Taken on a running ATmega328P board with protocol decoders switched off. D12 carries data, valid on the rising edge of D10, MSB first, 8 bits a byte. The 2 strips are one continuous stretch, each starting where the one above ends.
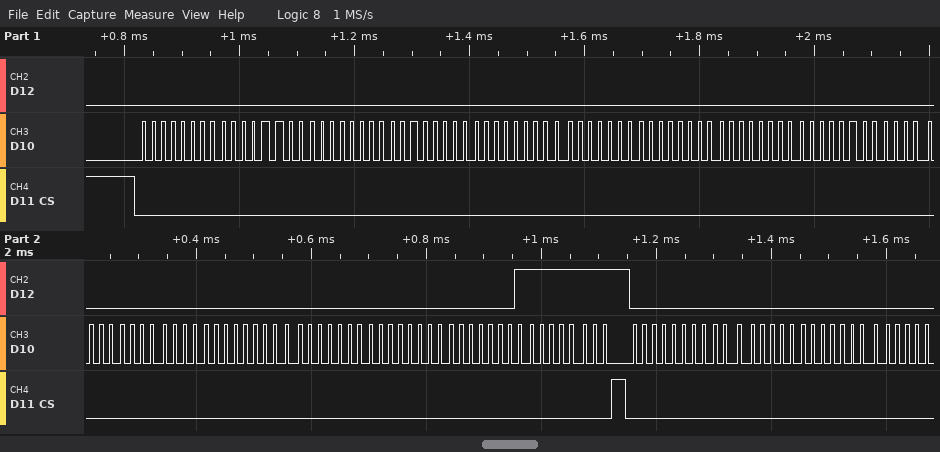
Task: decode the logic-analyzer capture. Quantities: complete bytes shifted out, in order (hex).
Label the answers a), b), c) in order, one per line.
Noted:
a) 00 00 00 00 00 00 00 00 00 00 00 00 00 00 01 FF 00 00 00
